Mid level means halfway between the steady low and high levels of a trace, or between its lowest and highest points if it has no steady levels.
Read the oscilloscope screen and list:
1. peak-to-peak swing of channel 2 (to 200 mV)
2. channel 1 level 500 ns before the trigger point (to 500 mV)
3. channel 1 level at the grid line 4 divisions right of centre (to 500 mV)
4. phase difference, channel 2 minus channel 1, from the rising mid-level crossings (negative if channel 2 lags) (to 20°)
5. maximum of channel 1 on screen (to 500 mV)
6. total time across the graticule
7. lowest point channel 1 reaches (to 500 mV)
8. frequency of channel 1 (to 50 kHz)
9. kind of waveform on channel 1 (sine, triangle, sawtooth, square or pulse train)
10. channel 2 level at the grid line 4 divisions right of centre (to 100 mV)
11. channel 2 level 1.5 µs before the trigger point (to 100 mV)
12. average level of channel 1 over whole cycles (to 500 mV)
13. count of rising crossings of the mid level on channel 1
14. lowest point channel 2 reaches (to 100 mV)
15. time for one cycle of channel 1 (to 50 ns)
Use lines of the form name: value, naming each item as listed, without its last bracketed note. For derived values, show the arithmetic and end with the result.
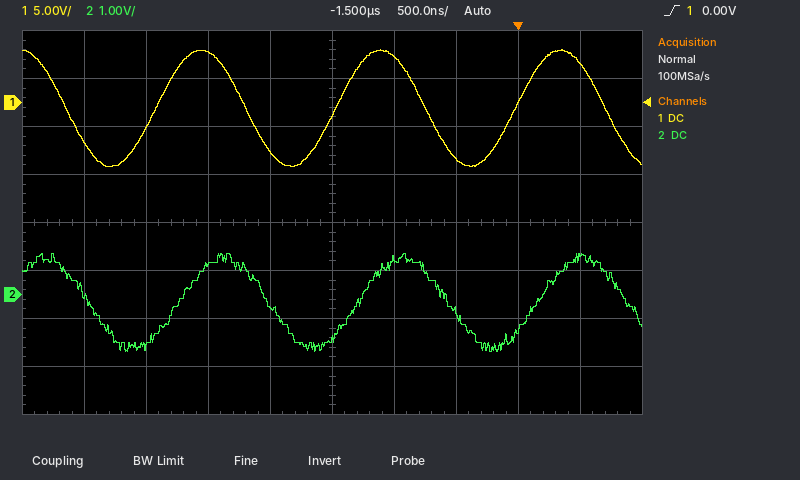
peak-to-peak swing of channel 2: 2.0 V
channel 1 level 500 ns before the trigger point: -6.0 V
channel 1 level at the grid line 4 divisions right of centre: 4.0 V
phase difference, channel 2 minus channel 1, from the rising mid-level crossings (negative if channel 2 lags): -40°
maximum of channel 1 on screen: 5.5 V
total time across the graticule: 5 µs
lowest point channel 1 reaches: -6.5 V
frequency of channel 1: 1 / 1.45 µs ≈ 690 kHz, so 700 kHz to the nearest 50 kHz
kind of waveform on channel 1: sine
channel 2 level at the grid line 4 divisions right of centre: 800 mV
channel 2 level 1.5 µs before the trigger point: -900 mV
average level of channel 1 over whole cycles: (5.5 V + (-6.5 V)) / 2 ≈ -500 mV
count of rising crossings of the mid level on channel 1: 3
lowest point channel 2 reaches: -1.2 V
time for one cycle of channel 1: 1.45 µs
